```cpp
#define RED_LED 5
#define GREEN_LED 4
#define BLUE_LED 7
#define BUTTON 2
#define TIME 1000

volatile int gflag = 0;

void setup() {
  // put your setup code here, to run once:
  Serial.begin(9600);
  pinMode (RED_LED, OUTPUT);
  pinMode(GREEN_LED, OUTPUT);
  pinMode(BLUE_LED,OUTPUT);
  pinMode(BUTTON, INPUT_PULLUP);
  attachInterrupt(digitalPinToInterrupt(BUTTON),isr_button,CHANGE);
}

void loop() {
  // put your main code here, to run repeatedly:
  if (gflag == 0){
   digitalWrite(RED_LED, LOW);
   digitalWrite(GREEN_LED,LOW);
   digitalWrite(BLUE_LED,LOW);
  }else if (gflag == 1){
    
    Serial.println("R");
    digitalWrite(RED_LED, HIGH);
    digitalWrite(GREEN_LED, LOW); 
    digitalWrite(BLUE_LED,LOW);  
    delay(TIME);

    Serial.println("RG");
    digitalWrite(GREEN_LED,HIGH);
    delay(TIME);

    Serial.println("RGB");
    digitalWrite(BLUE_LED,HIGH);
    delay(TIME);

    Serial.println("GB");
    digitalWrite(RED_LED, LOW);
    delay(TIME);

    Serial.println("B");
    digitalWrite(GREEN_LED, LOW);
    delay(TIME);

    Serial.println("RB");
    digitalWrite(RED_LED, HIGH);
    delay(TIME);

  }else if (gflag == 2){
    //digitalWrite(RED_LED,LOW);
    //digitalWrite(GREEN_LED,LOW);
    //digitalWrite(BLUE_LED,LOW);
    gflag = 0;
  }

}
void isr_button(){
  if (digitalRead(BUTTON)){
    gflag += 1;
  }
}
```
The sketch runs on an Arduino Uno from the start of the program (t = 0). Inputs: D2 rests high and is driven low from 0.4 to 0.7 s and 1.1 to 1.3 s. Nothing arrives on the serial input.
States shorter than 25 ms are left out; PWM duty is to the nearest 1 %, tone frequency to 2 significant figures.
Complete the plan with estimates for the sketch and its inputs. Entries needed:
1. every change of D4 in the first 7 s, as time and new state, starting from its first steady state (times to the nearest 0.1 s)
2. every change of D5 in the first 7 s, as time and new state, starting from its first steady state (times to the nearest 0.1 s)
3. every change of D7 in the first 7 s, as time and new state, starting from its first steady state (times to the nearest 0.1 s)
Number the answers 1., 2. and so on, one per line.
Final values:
1. 0 s low; 1.7 s high; 4.7 s low
2. 0 s low; 0.7 s high; 3.7 s low; 5.7 s high; 6.7 s low
3. 0 s low; 2.7 s high; 6.7 s low
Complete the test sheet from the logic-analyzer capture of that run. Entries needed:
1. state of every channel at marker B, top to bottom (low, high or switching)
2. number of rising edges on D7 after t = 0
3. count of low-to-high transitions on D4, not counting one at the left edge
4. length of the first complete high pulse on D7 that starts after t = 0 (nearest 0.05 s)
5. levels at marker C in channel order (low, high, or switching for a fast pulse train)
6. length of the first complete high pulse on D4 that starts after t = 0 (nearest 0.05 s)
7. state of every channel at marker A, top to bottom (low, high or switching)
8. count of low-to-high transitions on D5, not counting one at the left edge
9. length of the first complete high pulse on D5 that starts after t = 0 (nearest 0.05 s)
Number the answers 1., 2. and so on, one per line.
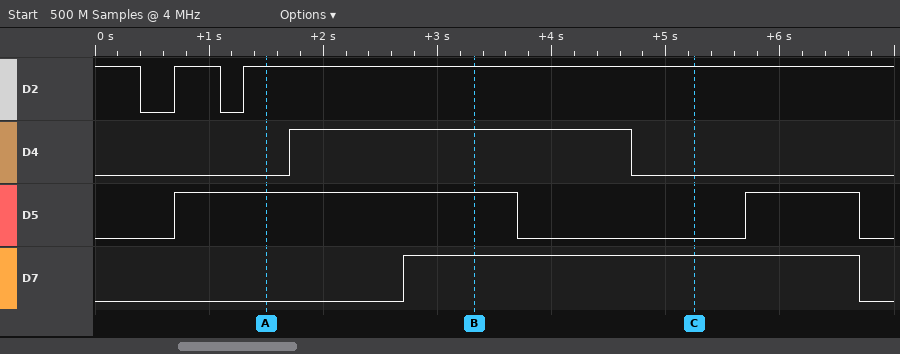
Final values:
1. D2 high, D4 high, D5 high, D7 high
2. 1
3. 1
4. 4.00 s
5. D2 high, D4 low, D5 low, D7 high
6. 3.00 s
7. D2 high, D4 low, D5 high, D7 low
8. 2
9. 3.00 s
